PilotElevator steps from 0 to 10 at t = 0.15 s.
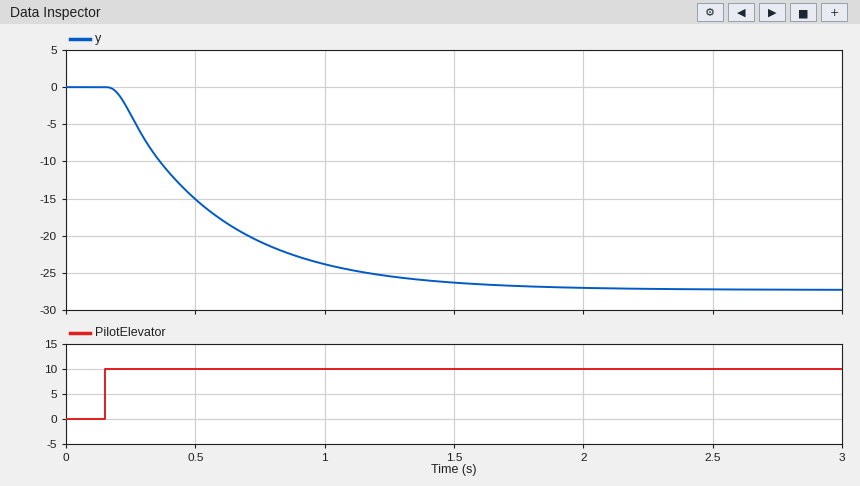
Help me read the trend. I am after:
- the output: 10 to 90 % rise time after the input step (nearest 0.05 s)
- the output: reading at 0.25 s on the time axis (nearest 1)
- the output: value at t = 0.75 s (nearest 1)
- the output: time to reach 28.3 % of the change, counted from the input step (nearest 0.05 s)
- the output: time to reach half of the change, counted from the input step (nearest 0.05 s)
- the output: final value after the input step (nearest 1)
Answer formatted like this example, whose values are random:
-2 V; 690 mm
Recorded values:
0.85 s; -4; -21; 0.15 s; 0.30 s; -27
